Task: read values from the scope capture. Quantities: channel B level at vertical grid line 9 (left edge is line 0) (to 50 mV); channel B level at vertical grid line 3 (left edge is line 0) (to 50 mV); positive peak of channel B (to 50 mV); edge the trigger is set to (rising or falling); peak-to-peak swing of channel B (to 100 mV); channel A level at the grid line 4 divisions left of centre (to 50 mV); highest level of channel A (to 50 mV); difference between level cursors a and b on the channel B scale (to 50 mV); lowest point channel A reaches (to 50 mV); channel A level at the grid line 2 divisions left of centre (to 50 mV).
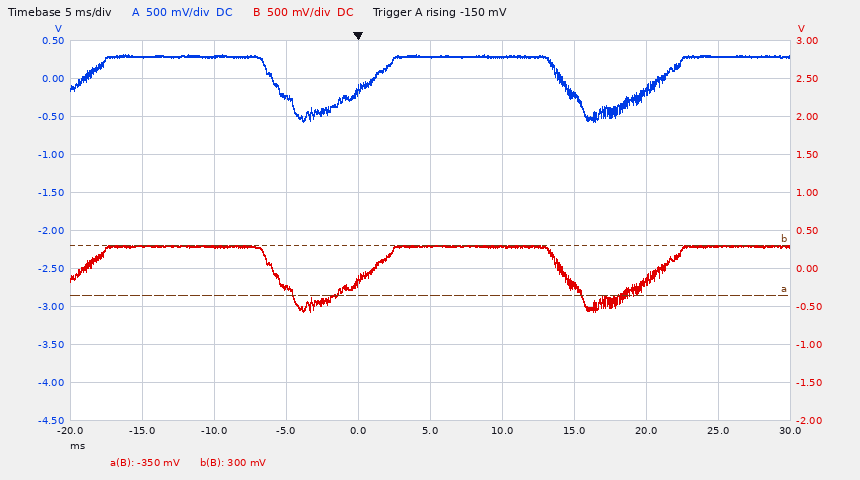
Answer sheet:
300 mV
-250 mV
300 mV
rising
900 mV
300 mV
300 mV
650 mV
-550 mV
-250 mV
